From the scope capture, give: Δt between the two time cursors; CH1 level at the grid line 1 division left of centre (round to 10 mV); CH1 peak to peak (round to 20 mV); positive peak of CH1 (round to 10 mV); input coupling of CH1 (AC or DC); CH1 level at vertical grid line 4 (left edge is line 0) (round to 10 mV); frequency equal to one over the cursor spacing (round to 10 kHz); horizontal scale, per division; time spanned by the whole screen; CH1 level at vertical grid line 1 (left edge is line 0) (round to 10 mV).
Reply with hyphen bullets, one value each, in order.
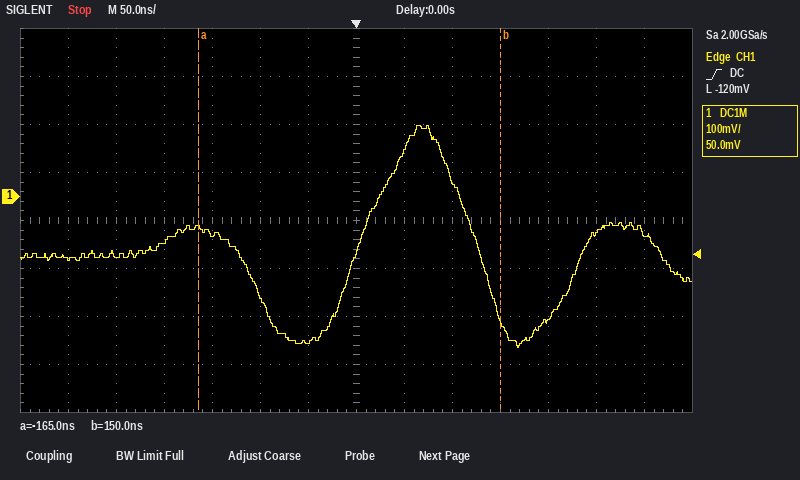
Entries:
- 315 ns
- -300 mV
- 460 mV
- 150 mV
- DC
- -80 mV
- 3.17 MHz
- 50 ns
- 700 ns
- -130 mV
